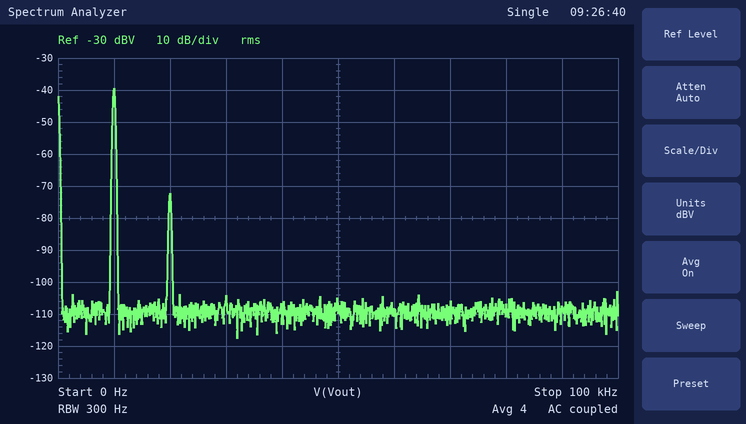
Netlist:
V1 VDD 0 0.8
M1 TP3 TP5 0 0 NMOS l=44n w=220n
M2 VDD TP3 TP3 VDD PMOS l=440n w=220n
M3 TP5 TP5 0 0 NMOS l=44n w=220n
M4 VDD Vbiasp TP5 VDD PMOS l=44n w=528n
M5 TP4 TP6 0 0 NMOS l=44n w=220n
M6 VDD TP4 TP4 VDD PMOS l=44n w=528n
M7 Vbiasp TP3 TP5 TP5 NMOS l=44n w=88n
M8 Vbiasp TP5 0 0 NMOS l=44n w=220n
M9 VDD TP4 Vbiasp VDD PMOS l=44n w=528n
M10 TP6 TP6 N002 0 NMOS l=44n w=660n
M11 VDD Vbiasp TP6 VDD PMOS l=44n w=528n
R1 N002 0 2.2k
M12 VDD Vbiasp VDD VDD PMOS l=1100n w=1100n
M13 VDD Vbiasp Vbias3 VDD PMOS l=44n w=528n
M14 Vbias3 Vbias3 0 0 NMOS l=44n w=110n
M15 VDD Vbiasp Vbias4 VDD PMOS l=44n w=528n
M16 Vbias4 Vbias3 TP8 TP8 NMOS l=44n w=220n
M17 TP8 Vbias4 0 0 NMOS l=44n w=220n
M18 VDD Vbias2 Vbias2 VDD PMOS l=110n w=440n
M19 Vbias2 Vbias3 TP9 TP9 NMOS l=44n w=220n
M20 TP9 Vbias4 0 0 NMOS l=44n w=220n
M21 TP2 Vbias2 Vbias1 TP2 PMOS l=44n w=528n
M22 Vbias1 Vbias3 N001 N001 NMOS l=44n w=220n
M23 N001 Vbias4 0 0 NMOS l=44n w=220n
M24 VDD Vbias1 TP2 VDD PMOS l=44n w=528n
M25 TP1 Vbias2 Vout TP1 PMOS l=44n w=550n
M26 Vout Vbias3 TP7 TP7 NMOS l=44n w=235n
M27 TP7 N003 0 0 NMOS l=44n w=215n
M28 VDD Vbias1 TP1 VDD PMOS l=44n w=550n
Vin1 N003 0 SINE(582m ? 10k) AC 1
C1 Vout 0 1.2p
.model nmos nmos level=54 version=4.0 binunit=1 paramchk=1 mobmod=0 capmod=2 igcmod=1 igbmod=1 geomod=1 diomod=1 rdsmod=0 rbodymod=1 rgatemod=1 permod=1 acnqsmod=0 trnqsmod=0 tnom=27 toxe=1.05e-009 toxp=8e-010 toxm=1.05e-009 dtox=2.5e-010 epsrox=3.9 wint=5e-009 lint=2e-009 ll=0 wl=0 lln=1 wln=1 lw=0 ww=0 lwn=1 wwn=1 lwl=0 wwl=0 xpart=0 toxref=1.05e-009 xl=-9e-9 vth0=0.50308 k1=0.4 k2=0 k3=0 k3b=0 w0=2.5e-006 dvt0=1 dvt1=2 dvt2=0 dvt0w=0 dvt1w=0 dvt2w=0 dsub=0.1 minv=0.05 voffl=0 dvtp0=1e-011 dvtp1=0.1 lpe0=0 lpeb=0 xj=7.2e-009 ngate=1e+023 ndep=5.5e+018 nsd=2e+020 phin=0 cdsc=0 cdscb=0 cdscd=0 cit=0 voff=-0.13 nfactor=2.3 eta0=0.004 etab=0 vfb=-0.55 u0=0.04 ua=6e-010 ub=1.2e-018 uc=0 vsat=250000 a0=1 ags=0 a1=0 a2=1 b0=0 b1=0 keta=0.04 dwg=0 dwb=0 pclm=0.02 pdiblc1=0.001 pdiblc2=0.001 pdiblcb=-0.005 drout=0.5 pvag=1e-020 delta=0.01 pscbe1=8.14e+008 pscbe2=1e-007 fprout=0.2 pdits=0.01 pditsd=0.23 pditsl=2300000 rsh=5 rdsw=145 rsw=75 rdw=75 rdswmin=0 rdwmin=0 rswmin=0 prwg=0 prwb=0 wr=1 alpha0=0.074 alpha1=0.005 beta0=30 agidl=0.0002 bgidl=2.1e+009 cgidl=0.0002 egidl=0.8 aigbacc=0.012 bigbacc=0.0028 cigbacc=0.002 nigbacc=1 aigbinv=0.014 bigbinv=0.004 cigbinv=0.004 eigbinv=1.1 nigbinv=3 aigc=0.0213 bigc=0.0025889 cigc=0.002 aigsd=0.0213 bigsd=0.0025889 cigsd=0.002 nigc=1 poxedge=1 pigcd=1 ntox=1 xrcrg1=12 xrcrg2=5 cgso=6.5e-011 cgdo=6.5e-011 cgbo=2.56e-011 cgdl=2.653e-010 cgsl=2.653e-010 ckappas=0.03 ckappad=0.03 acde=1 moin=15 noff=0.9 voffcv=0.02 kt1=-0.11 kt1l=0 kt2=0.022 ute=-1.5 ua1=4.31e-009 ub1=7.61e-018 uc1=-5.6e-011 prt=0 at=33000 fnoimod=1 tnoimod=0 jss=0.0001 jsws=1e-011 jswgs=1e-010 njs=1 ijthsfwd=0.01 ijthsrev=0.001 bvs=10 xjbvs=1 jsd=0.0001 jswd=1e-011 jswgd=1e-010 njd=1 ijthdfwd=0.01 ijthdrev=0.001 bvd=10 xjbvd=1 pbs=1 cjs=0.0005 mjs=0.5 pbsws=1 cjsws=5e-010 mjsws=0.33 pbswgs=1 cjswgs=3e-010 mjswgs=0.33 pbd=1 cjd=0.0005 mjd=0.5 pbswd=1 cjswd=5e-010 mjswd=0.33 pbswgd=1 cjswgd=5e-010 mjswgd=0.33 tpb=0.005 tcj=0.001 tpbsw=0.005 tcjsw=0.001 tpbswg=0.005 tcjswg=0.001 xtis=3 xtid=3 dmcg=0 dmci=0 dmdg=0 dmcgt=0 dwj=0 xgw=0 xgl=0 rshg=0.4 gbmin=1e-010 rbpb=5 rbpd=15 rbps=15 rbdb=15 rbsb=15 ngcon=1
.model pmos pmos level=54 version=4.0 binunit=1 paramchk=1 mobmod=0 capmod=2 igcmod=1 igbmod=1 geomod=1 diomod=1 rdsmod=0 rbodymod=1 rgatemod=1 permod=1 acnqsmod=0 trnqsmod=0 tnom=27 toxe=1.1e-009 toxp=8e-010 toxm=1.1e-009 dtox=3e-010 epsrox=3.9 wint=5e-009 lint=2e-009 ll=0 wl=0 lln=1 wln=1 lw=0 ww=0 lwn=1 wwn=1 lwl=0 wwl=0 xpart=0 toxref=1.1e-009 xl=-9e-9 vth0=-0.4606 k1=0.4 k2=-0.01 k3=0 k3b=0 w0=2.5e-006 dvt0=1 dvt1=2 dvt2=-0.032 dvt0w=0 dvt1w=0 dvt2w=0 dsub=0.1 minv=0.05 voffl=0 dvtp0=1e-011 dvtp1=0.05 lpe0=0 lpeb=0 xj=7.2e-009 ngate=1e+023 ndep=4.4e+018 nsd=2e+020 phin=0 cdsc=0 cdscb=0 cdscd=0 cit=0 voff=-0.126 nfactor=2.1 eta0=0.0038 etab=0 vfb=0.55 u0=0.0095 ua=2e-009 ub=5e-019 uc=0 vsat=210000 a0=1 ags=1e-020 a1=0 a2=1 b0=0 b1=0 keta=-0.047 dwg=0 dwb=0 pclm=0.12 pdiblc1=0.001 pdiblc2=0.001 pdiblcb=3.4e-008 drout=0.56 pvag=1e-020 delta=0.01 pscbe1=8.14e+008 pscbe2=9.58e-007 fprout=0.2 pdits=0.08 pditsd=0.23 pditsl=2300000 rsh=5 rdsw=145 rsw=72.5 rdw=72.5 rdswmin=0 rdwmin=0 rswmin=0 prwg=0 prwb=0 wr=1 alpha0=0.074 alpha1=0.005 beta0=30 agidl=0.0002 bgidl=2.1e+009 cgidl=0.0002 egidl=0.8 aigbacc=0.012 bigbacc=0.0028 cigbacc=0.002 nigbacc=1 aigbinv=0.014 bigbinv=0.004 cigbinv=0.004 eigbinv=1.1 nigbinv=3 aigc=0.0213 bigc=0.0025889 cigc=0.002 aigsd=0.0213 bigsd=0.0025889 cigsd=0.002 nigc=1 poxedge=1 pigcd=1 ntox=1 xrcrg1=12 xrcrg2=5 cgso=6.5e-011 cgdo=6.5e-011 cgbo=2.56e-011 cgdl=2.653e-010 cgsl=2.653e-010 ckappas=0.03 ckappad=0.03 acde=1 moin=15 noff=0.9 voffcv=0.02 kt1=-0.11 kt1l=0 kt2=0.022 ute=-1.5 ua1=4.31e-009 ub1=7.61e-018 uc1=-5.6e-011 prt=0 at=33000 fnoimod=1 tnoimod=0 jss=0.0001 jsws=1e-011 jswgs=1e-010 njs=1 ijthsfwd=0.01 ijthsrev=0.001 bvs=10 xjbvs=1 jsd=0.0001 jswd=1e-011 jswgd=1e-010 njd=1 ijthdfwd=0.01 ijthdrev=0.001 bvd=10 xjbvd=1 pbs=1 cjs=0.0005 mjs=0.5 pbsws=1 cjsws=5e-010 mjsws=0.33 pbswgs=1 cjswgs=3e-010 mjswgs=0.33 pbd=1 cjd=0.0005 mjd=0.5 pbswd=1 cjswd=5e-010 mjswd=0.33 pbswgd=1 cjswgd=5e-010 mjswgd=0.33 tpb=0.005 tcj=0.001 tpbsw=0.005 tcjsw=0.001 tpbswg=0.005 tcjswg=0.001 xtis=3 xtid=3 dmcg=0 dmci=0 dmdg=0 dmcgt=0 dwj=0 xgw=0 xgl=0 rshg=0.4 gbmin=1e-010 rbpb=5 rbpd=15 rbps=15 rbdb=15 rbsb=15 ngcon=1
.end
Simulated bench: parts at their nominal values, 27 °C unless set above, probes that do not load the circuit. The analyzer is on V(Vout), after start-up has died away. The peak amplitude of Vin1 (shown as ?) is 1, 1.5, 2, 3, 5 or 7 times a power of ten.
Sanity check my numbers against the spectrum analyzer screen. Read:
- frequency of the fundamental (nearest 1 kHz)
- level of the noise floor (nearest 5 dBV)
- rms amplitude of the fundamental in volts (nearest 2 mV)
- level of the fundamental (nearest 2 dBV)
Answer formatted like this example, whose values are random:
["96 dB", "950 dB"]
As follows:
["10 kHz", "-110 dBV", "10 mV", "-40 dBV"]
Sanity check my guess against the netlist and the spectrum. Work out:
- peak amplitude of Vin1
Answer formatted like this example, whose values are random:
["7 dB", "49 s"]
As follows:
["7 mV"]
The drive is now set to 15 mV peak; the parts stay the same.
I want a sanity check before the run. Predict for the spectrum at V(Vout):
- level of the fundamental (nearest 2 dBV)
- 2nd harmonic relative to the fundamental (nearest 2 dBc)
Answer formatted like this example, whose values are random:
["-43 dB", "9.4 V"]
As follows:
["-32 dBV", "-26 dBc"]
